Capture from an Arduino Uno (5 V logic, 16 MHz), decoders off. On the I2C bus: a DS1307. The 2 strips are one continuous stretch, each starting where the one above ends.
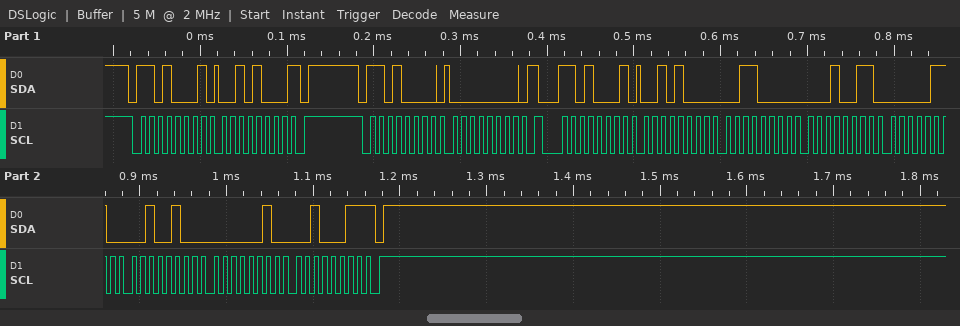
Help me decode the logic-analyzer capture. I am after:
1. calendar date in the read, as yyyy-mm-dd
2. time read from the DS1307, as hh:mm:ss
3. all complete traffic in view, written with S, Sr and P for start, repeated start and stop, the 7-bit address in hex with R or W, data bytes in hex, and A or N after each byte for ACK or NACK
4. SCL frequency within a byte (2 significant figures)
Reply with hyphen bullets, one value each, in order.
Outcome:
- 2023-02-24
- 13:30:28
- S 68R A 28 N P S 68W A 00 A Sr 68R A 28 A 30 A 13 A 06 A 24 A 02 A 23 N P
- 100 kHz
